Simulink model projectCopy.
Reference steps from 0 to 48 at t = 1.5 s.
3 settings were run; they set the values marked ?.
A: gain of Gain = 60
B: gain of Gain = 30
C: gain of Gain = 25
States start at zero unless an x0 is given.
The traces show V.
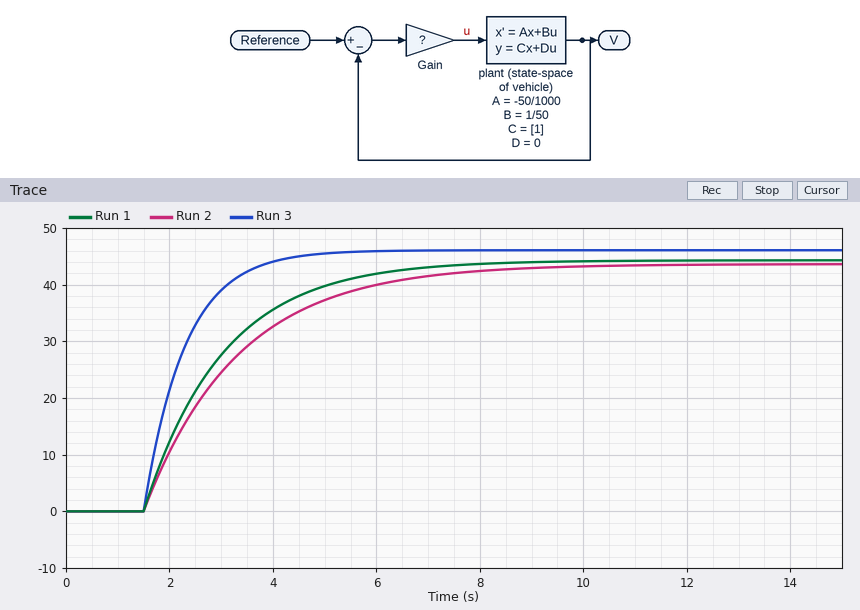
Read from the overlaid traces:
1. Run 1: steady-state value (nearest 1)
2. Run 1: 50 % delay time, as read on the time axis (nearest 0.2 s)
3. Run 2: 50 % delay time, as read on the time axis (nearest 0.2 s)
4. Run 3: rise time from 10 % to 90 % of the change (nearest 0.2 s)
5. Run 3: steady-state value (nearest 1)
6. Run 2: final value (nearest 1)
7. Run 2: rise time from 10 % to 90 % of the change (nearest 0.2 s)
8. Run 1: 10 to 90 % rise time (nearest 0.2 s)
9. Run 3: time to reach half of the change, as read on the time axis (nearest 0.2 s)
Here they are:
44
2.6 s
2.8 s
1.8 s
46
44
4.0 s
3.4 s
2.0 s
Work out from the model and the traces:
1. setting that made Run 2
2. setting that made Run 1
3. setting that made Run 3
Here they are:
C
B
A
